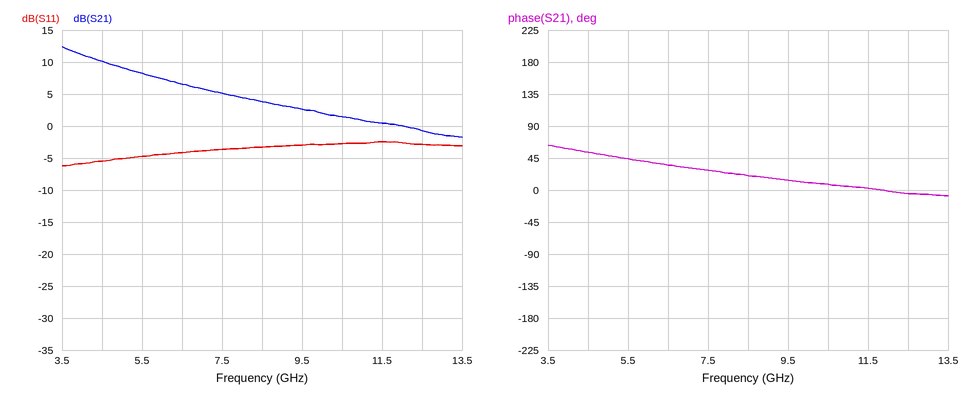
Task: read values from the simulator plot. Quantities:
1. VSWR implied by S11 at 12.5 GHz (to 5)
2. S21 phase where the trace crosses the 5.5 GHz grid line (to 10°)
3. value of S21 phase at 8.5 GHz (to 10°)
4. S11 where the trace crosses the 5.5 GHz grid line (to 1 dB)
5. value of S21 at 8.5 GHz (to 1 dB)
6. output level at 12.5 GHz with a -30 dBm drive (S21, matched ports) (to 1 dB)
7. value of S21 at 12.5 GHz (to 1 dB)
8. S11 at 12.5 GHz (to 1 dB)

5
40°
20°
-5 dB
4 dB
-31 dBm
-1 dB
-3 dB
